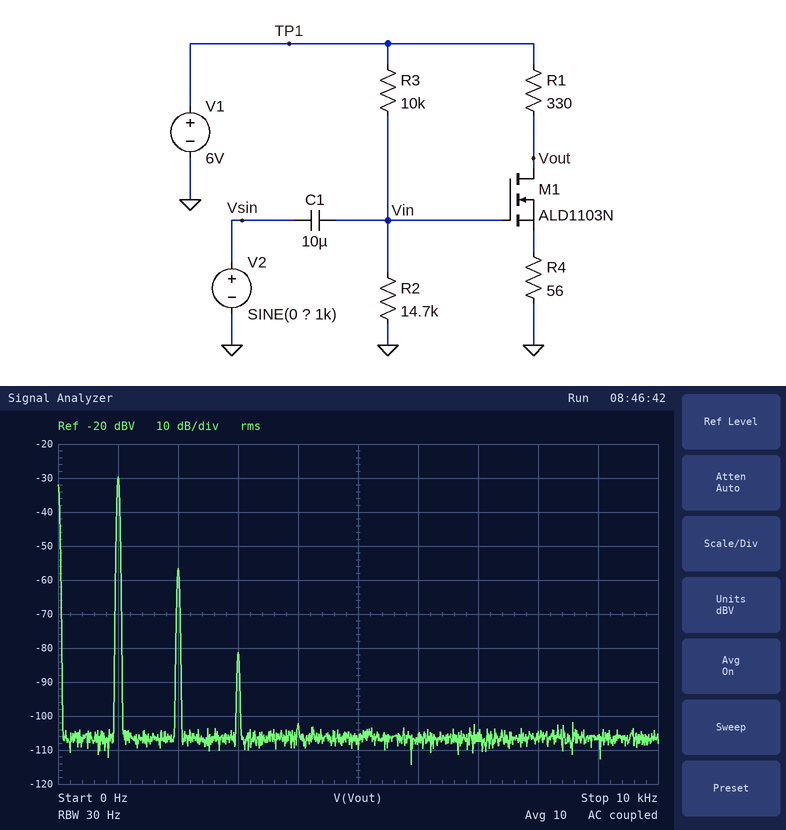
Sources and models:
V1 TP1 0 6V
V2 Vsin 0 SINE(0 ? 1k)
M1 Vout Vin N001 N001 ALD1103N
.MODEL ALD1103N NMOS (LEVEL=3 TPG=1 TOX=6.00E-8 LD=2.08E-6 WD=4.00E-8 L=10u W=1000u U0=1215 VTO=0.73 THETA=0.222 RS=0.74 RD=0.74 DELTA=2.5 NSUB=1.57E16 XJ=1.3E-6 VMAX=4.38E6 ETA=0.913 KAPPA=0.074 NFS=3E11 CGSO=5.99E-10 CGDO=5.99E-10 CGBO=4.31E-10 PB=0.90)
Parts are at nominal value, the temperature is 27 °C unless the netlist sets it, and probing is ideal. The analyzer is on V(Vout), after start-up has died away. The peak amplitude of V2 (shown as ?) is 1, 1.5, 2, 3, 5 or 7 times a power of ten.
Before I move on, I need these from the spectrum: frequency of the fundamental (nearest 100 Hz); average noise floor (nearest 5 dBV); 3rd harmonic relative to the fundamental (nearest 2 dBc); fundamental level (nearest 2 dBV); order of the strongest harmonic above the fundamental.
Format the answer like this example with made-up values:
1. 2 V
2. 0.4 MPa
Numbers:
1. 1.0 kHz
2. -105 dBV
3. -52 dBc
4. -30 dBV
5. 2
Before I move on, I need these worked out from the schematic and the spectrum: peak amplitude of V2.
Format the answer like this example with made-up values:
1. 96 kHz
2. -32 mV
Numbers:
1. 70 mV
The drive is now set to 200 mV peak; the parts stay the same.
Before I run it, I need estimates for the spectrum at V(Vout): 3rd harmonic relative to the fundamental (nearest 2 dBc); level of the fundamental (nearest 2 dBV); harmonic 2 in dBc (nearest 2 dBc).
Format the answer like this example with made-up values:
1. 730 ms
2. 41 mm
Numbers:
1. -32 dBc
2. -20 dBV
3. -18 dBc
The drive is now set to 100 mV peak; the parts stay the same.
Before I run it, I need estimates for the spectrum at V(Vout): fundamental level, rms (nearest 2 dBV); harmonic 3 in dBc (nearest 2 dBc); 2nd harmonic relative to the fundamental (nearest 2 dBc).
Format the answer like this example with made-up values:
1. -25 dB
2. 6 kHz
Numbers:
1. -26 dBV
2. -46 dBc
3. -24 dBc
